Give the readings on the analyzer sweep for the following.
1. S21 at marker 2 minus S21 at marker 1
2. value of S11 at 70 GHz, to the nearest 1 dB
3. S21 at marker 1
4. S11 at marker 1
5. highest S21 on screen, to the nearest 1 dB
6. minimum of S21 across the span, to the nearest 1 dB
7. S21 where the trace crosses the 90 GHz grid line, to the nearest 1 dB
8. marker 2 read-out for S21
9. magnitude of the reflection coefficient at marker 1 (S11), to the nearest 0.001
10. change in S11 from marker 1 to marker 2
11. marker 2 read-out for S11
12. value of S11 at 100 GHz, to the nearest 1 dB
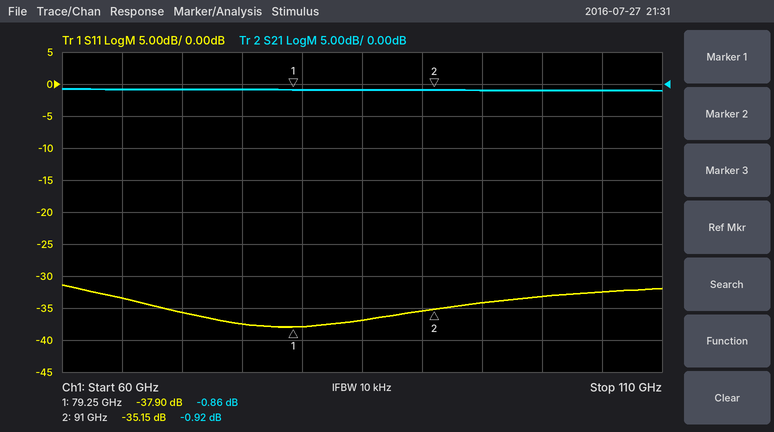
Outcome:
-0.06 dB
-36 dB
-0.86 dB
-37.90 dB
-1 dB
-1 dB
-1 dB
-0.92 dB
0.013
2.75 dB
-35.15 dB
-33 dB
